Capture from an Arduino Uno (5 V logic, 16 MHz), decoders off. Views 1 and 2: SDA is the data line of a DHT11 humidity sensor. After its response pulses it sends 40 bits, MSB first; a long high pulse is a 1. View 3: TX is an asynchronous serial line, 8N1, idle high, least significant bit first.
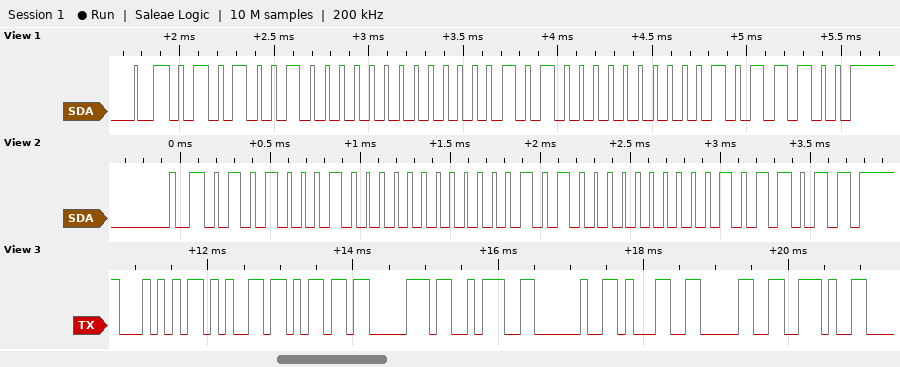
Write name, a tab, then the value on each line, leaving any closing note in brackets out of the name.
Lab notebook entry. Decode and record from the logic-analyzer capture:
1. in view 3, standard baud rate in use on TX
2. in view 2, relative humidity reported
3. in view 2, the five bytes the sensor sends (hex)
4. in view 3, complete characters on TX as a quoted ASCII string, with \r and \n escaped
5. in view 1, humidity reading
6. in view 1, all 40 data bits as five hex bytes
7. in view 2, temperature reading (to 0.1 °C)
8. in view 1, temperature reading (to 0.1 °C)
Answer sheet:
in view 3, standard baud rate in use on TX	9600 baud
in view 2, relative humidity reported	81 %
in view 2, the five bytes the sensor sends	51 00 0A 00 5B
in view 3, complete characters on TX as a quoted ASCII string, with \r and \n escaped	"Temp: 10."
in view 1, humidity reading	82 %
in view 1, all 40 data bits as five hex bytes	52 00 0A 00 5C
in view 2, temperature reading	10.0 °C
in view 1, temperature reading	10.0 °C
